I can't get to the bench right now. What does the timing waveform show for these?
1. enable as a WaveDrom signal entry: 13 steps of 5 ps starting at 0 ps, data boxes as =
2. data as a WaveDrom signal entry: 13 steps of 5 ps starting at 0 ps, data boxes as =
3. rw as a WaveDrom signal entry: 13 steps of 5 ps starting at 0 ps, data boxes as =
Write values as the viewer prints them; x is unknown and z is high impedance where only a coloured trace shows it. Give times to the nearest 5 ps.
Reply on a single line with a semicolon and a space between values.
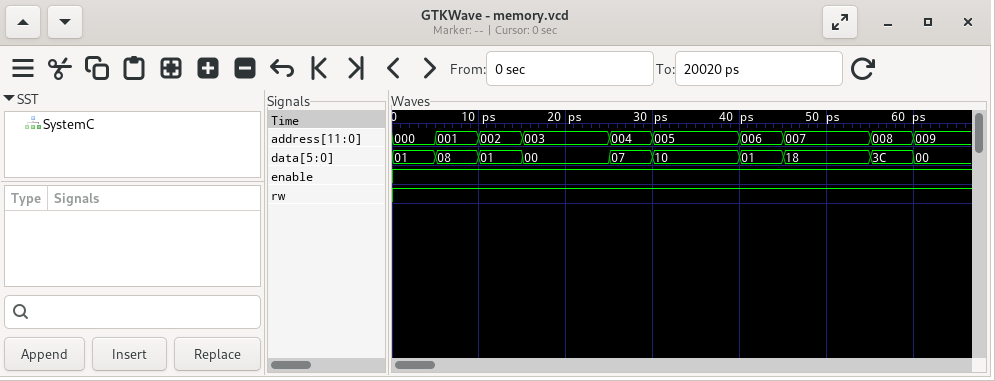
{name: 'enable', wave: '1............'}; {name: 'data', wave: '====.==.==.==', data: '01 08 01 00 07 10 01 18 3C 00'}; {name: 'rw', wave: '1............'}
